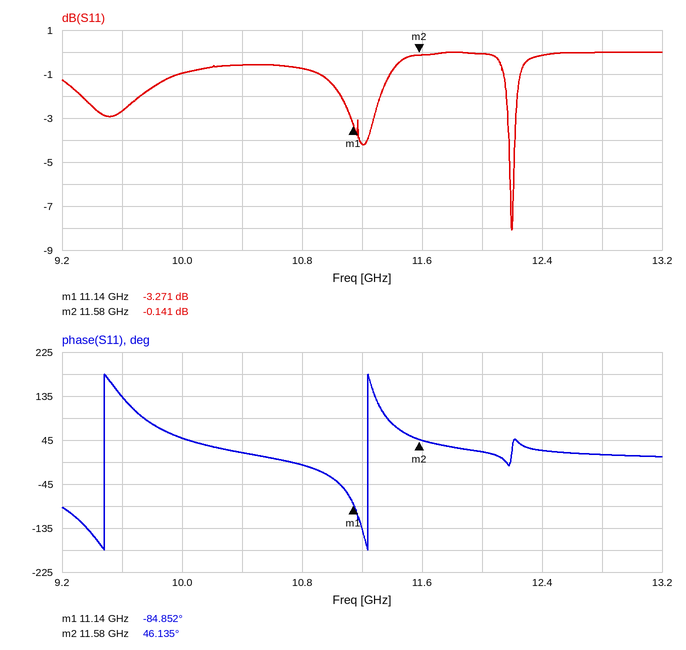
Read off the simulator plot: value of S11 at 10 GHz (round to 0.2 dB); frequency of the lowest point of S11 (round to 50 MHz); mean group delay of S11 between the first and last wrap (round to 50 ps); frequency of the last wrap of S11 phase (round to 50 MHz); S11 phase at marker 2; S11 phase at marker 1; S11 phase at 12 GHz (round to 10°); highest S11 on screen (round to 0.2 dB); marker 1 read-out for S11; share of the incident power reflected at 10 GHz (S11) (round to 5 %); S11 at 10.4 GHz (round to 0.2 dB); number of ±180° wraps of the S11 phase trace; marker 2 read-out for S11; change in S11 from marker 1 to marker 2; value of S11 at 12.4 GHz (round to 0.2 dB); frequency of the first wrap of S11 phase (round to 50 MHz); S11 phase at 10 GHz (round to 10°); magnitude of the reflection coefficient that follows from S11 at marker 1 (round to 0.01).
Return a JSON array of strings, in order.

["-1.0 dB", "12.20 GHz", "550 ps", "11.25 GHz", "46.135°", "-84.852°", "20°", "0.0 dB", "-3.271 dB", "80 %", "-0.6 dB", "2", "-0.141 dB", "3.130 dB", "-0.2 dB", "9.50 GHz", "50°", "0.69"]
